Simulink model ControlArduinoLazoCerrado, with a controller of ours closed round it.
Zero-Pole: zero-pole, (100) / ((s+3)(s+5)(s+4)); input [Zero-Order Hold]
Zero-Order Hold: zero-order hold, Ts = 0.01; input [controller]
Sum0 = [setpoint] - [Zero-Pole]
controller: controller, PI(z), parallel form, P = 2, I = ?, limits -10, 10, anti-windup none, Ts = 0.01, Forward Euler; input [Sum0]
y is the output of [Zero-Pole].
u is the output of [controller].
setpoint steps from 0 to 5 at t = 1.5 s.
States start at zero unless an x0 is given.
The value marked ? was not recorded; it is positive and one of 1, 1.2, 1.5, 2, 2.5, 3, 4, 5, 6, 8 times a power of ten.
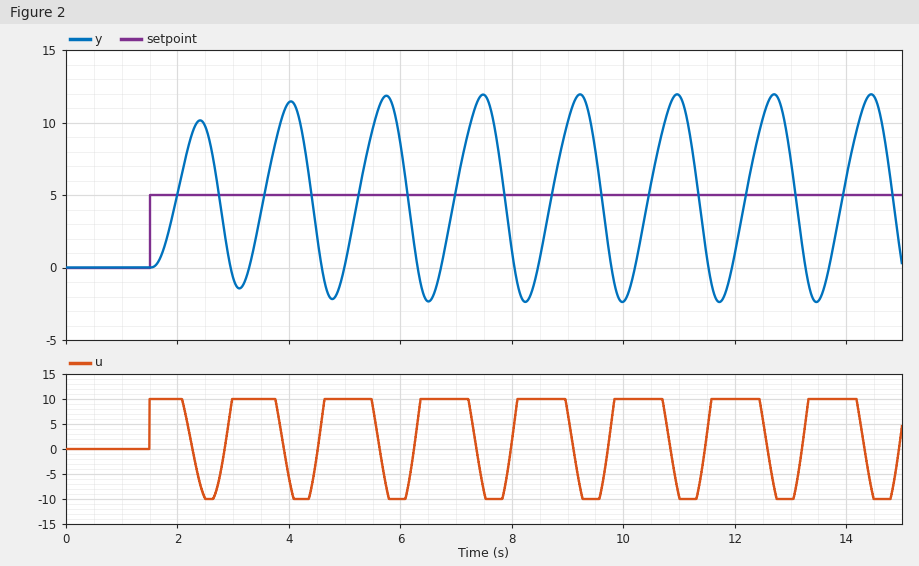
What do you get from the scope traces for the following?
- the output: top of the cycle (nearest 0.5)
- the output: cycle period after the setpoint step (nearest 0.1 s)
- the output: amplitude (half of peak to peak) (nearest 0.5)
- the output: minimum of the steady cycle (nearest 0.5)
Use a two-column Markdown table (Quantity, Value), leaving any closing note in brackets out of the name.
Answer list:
| Quantity | Value |
|---|---|
| the output: top of the cycle | 12.0 |
| the output: cycle period after the setpoint step | 1.7 s |
| the output: amplitude (half of peak to peak) | 7.0 |
| the output: minimum of the steady cycle | -2.5 |
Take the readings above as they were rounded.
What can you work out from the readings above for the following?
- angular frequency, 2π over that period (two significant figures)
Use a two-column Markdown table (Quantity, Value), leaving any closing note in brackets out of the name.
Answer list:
| Quantity | Value |
|---|---|
| angular frequency, 2π over that period | 3.7 rad/s |
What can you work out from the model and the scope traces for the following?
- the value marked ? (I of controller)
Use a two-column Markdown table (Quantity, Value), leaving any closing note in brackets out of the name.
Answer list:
| Quantity | Value |
|---|---|
| the value marked ? | 8 |
